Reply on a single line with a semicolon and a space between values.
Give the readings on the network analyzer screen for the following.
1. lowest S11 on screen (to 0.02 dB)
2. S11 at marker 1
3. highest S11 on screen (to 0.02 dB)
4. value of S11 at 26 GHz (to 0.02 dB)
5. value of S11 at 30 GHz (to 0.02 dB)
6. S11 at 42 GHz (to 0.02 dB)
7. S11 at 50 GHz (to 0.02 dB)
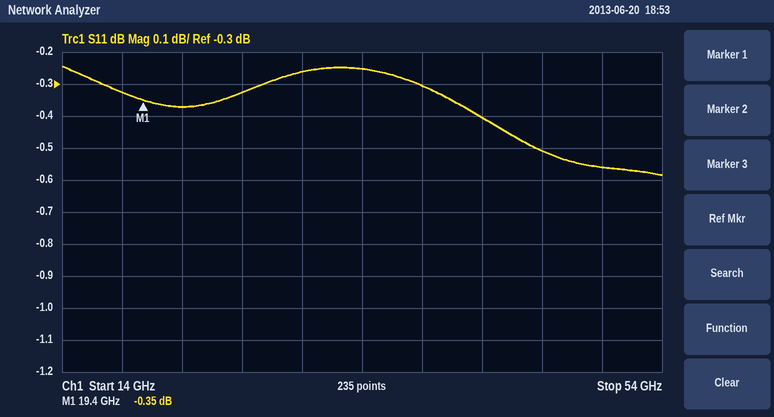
-0.58 dB; -0.35 dB; -0.24 dB; -0.32 dB; -0.26 dB; -0.40 dB; -0.56 dB
